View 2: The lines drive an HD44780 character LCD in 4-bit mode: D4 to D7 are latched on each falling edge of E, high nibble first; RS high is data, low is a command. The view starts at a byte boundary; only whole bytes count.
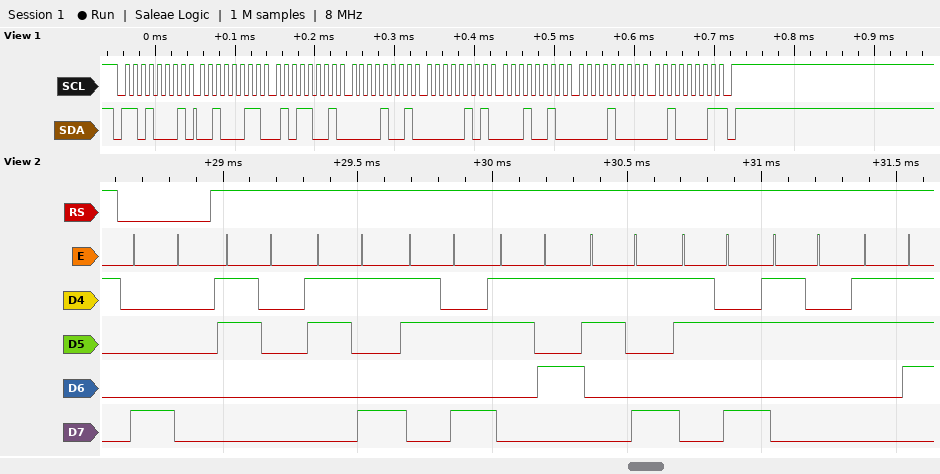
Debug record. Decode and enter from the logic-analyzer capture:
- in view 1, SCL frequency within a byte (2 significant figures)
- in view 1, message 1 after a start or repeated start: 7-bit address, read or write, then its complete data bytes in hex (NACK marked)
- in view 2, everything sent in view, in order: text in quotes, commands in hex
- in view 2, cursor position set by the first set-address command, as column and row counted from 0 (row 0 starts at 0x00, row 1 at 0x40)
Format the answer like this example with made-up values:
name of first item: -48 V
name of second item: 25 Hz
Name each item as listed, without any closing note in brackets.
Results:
in view 1, SCL frequency within a byte: 100 kHz
in view 1, message 1 after a start or repeated start: 7-bit address, read or write, then its complete data bytes in hex: 0x68 read: 23 59 09 05 12 08 21 NACK
in view 2, everything sent in view, in order: text in quotes, commands in hex: 0x80 "09:59:27"
in view 2, cursor position set by the first set-address command, as column and row counted from 0: column 0, row 0
